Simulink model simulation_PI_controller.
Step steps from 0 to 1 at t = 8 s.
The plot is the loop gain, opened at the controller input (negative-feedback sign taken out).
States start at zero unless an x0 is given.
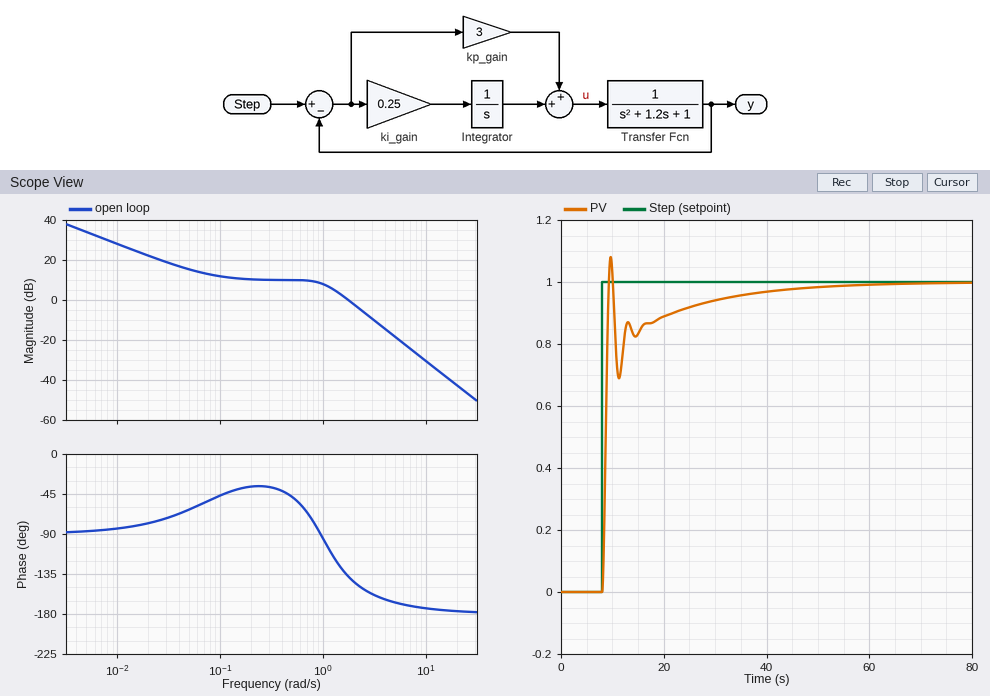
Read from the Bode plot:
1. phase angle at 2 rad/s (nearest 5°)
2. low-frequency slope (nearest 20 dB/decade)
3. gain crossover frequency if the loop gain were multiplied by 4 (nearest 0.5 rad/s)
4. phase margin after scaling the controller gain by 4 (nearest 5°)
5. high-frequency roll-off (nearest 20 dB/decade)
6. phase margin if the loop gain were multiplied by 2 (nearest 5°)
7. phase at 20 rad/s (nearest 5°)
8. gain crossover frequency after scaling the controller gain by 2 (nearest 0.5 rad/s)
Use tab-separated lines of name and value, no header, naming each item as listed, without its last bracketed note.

phase angle at 2 rad/s	-145°
low-frequency slope	-20 dB/decade
gain crossover frequency if the loop gain were multiplied by 4	3.5 rad/s
phase margin after scaling the controller gain by 4	20°
high-frequency roll-off	-40 dB/decade
phase margin if the loop gain were multiplied by 2	30°
phase at 20 rad/s	-175°
gain crossover frequency after scaling the controller gain by 2	2.5 rad/s
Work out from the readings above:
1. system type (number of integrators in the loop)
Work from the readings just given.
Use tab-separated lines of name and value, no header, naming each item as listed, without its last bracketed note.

system type	1
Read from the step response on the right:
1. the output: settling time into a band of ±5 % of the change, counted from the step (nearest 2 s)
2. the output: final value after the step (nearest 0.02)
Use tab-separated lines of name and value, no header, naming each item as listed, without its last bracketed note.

the output: settling time into a band of ±5 % of the change, counted from the step	24 s
the output: final value after the step	1.00
